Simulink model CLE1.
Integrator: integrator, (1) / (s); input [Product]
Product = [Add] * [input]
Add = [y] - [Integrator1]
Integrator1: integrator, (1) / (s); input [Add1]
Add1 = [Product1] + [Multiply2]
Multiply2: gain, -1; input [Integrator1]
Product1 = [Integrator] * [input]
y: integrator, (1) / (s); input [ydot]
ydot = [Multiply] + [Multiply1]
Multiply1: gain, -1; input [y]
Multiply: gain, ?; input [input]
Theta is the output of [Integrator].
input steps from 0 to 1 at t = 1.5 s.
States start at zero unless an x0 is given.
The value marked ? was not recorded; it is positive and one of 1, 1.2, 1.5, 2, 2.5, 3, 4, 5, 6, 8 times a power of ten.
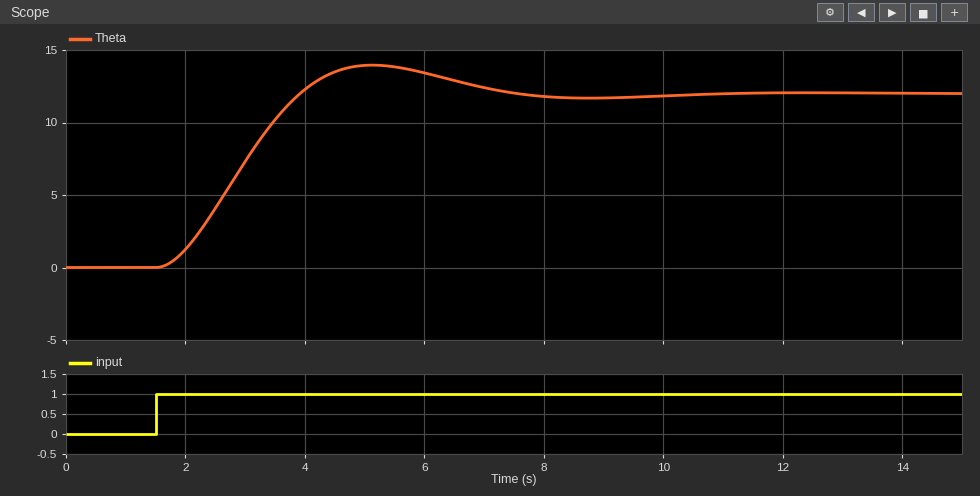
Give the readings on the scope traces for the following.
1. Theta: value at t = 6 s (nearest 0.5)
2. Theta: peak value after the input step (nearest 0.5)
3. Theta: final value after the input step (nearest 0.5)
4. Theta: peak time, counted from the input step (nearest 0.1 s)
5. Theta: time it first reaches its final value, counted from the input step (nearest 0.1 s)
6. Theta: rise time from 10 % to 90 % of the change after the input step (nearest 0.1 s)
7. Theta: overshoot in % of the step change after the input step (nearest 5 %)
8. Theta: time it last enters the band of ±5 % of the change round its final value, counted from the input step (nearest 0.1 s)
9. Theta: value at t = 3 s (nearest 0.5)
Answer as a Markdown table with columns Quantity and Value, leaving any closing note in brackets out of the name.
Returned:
| Quantity | Value |
|---|---|
| Theta: value at t = 6 s | 13.5 |
| Theta: peak value after the input step | 14.0 |
| Theta: final value after the input step | 12.0 |
| Theta: peak time, counted from the input step | 3.6 s |
| Theta: time it first reaches its final value, counted from the input step | 2.4 s |
| Theta: rise time from 10 % to 90 % of the change after the input step | 1.6 s |
| Theta: overshoot in % of the step change after the input step | 15 % |
| Theta: time it last enters the band of ±5 % of the change round its final value, counted from the input step | 5.3 s |
| Theta: value at t = 3 s | 7.5 |
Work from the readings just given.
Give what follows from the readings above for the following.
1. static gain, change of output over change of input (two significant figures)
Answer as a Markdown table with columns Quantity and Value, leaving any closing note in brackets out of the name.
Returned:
| Quantity | Value |
|---|---|
| static gain, change of output over change of input | 12 |
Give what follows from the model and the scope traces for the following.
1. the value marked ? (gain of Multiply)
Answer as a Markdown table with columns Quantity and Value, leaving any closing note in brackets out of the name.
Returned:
| Quantity | Value |
|---|---|
| the value marked ? | 12 |
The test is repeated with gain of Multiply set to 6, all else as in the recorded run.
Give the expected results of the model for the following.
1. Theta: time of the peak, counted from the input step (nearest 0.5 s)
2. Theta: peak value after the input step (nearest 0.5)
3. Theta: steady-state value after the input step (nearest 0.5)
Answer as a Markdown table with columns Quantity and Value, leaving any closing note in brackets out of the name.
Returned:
| Quantity | Value |
|---|---|
| Theta: time of the peak, counted from the input step | 3.5 s |
| Theta: peak value after the input step | 7.0 |
| Theta: steady-state value after the input step | 6.0 |
